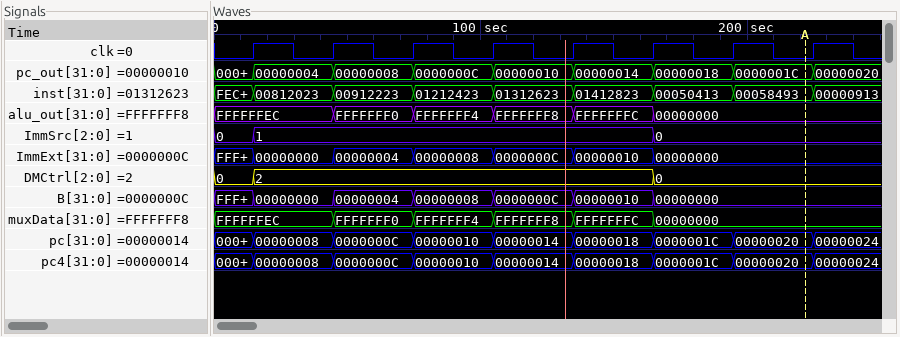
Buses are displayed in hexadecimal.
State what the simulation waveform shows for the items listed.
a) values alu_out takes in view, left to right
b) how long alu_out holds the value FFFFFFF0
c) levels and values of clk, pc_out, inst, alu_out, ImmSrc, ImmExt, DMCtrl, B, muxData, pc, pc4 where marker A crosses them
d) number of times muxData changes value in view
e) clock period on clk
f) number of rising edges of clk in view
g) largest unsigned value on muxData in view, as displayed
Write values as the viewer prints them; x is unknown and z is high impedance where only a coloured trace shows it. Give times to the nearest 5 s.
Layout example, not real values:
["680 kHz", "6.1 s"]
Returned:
["FFFFFFEC, FFFFFFF0, FFFFFFF4, FFFFFFF8, FFFFFFFC, 00000000", "30 s", "clk=0, pc_out=0000001C, inst=00058493, alu_out=00000000, ImmSrc=0, ImmExt=00000000, DMCtrl=0, B=00000000, muxData=00000000, pc=00000020, pc4=00000020", "5", "30 s", "8", "FFFFFFFC"]
